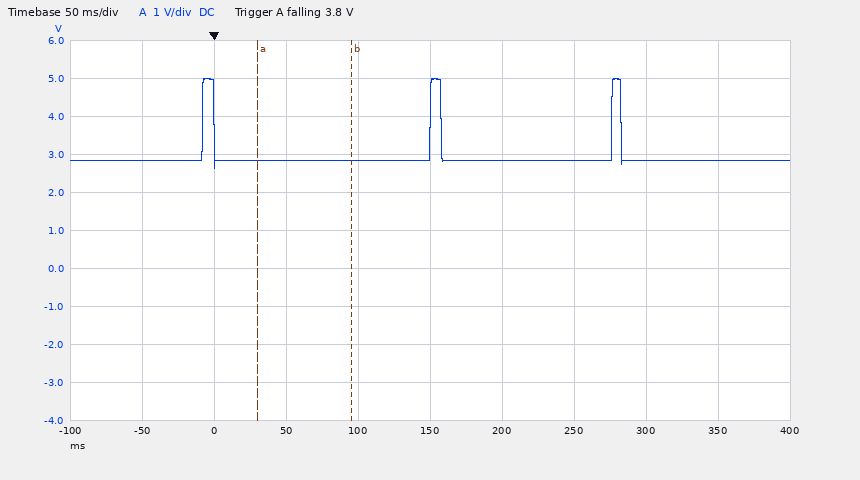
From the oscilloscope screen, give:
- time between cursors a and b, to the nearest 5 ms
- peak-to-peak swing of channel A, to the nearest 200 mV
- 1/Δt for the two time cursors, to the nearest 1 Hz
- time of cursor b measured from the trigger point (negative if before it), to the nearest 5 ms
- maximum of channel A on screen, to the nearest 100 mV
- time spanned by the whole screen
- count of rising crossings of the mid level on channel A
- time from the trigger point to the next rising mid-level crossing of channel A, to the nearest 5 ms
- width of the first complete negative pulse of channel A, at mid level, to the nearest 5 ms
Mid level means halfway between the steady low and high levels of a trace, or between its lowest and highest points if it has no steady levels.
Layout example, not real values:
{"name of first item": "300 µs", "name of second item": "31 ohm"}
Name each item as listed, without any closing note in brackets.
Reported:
{"time between cursors a and b, to the nearest 5 ms": "65 ms", "peak-to-peak swing of channel A, to the nearest 200 mV": "2.4 V", "1/Δt for the two time cursors, to the nearest 1 Hz": "15 Hz", "time of cursor b measured from the trigger point (negative if before it), to the nearest 5 ms": "+95 ms", "maximum of channel A on screen, to the nearest 100 mV": "5.0 V", "time spanned by the whole screen": "500 ms", "count of rising crossings of the mid level on channel A": "3", "time from the trigger point to the next rising mid-level crossing of channel A, to the nearest 5 ms": "150 ms", "width of the first complete negative pulse of channel A, at mid level, to the nearest 5 ms": "150 ms"}
